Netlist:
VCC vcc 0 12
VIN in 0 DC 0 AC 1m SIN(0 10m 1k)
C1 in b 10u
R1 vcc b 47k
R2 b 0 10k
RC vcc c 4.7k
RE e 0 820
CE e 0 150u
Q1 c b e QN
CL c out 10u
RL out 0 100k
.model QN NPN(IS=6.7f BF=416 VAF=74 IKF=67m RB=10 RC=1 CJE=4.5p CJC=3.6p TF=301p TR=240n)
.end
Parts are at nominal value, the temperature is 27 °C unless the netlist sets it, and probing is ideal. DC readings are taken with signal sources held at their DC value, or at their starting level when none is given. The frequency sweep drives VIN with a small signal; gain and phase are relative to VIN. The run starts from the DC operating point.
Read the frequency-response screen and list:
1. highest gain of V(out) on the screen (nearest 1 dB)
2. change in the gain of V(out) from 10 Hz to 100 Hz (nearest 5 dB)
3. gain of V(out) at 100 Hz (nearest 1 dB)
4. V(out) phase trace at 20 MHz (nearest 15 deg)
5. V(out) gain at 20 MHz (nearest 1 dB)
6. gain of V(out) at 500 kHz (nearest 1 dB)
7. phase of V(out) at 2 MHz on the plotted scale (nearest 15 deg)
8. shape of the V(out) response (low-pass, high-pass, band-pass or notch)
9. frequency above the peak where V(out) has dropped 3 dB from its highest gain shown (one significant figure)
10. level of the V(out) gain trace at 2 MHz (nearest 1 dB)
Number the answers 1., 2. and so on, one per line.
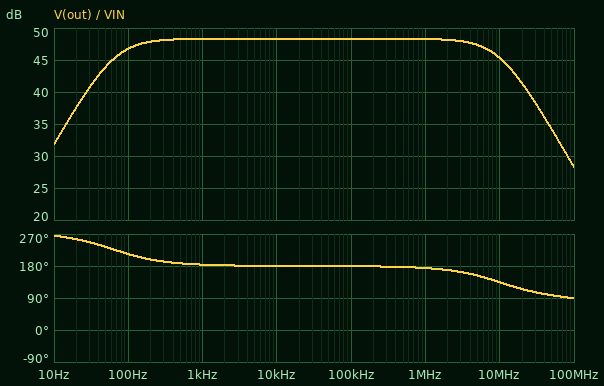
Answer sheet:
1. 48 dB
2. 15 dB
3. 47 dB
4. 120 deg
5. 41 dB
6. 48 dB
7. 165 deg
8. band-pass
9. 10 MHz
10. 48 dB
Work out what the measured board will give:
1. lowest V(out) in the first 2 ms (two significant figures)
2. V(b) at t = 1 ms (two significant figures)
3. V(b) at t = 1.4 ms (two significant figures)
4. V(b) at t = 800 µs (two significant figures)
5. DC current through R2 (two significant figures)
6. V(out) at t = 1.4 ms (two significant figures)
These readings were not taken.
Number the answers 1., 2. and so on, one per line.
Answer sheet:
1. -2.5 V
2. 2.1 V
3. 2.1 V
4. 2.1 V
5. 210 µA
6. -1.2 V
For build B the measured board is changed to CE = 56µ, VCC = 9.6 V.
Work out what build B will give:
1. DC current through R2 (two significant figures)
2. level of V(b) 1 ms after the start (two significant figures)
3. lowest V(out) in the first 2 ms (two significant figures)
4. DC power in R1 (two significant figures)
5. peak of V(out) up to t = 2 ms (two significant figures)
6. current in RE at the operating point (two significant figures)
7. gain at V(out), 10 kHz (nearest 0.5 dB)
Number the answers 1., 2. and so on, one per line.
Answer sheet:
1. 170 µA
2. 1.7 V
3. -2.0 V
4. 1.3 mW
5. 1.8 V
6. 1.2 mA
7. 45.5 dB
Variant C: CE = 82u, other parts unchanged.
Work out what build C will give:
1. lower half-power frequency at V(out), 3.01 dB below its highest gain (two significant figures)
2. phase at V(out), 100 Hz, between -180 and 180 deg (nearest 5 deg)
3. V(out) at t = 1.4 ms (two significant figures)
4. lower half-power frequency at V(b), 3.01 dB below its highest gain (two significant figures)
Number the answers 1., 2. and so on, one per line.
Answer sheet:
1. 120 Hz
2. -130 deg
3. -1.1 V
4. 2.0 Hz
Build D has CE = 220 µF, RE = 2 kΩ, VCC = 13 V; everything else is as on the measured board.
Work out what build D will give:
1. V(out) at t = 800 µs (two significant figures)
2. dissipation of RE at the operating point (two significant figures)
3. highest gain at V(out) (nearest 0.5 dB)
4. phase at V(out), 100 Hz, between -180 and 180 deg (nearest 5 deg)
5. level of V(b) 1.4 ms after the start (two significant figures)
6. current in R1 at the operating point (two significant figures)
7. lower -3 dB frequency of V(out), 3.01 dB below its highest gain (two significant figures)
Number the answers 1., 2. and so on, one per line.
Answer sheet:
1. 1.1 V
2. 1.3 mW
3. 42.5 dB
4. -165 deg
5. 2.3 V
6. 230 µA
7. 23 Hz
